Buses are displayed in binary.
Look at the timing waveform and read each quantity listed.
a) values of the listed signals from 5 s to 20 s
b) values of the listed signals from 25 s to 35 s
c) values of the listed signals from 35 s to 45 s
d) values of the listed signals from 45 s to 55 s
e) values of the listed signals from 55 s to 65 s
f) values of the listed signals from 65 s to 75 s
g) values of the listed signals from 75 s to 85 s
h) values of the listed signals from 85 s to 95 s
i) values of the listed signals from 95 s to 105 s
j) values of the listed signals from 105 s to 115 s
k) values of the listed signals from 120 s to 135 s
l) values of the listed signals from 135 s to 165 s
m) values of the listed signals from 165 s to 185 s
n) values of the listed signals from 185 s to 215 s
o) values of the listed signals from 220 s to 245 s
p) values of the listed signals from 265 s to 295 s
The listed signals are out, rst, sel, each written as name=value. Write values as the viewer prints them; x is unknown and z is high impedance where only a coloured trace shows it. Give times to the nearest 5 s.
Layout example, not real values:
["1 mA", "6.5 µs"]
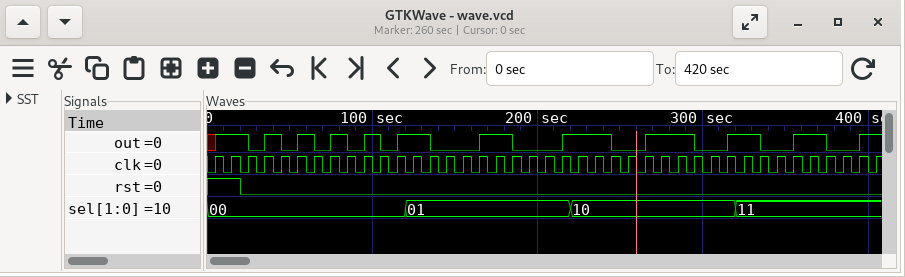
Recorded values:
["out=1, rst=1, sel=00", "out=0, rst=0, sel=00", "out=1, rst=0, sel=00", "out=0, rst=0, sel=00", "out=1, rst=0, sel=00", "out=0, rst=0, sel=00", "out=1, rst=0, sel=00", "out=0, rst=0, sel=00", "out=1, rst=0, sel=00", "out=0, rst=0, sel=00", "out=1, rst=0, sel=01", "out=0, rst=0, sel=01", "out=1, rst=0, sel=01", "out=0, rst=0, sel=01", "out=1, rst=0, sel=10", "out=1, rst=0, sel=10"]
